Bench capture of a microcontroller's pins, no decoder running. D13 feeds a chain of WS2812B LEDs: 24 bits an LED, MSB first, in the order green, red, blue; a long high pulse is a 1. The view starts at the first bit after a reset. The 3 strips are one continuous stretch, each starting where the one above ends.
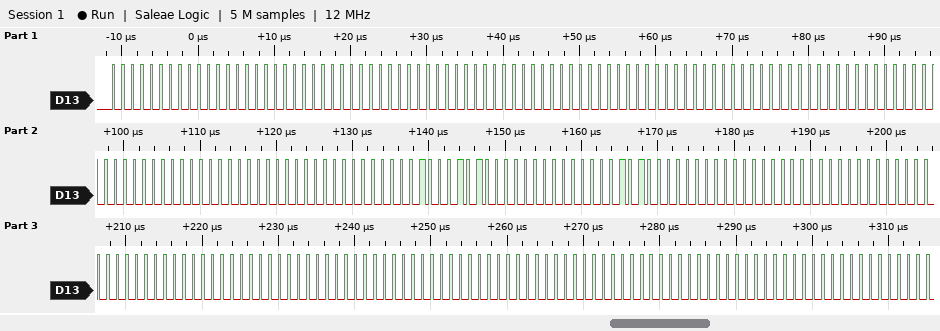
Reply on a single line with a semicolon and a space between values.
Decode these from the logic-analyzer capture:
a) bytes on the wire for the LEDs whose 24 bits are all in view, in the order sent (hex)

00 00 00 00 00 00 00 00 00 00 00 00 00 00 00 8A 00 05 00 00 00 00 00 00 00 00 00 00 00 00
